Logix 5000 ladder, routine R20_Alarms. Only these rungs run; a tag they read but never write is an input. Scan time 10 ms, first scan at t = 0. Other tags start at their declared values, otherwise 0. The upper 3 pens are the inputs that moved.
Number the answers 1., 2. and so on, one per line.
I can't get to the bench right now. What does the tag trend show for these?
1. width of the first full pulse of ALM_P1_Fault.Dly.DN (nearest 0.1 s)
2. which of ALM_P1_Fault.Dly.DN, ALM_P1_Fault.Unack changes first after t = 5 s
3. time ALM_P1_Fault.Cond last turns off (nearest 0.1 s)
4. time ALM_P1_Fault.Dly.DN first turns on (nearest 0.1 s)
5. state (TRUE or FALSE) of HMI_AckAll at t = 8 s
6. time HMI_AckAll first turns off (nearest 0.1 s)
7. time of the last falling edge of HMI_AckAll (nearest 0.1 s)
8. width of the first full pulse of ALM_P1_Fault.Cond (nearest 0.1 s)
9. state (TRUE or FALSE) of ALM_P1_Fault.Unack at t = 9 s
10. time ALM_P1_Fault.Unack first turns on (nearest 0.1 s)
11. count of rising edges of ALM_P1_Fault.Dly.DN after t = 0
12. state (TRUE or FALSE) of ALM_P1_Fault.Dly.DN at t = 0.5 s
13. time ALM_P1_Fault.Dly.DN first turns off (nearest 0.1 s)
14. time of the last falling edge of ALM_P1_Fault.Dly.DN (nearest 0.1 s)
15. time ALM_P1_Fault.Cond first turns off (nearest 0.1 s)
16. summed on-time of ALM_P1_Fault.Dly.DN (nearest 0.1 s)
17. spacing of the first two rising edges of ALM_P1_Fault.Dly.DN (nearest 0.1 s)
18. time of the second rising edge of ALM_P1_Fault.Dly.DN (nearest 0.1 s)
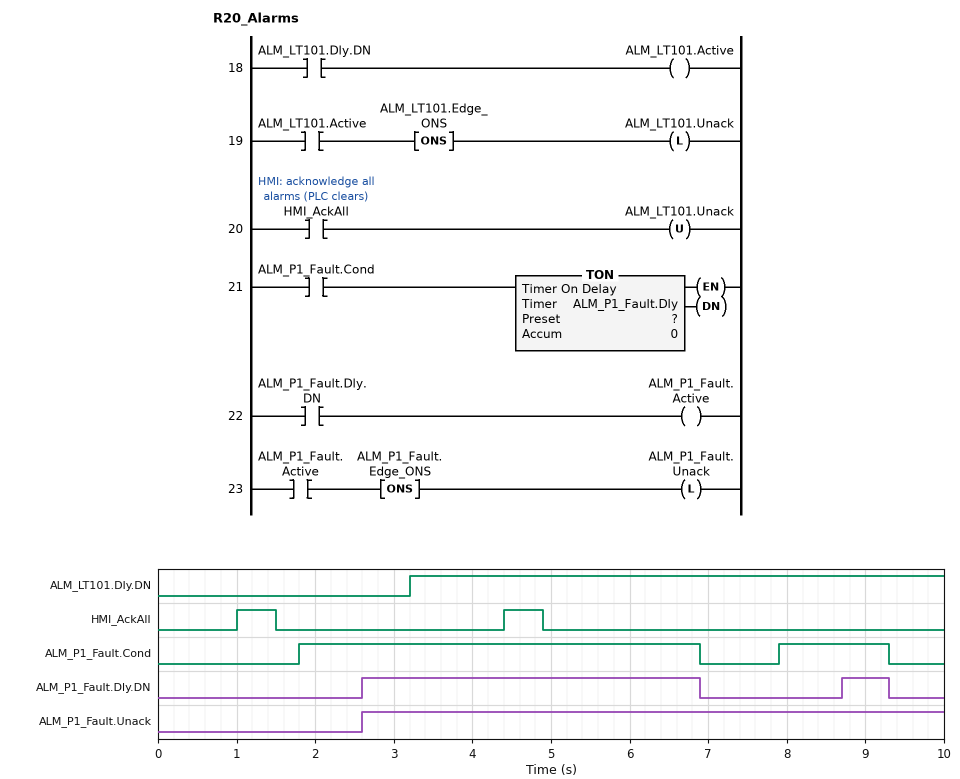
1. 4.3 s
2. ALM_P1_Fault.Dly.DN
3. 9.3 s
4. 2.6 s
5. FALSE
6. 1.5 s
7. 4.9 s
8. 5.1 s
9. TRUE
10. 2.6 s
11. 2
12. FALSE
13. 6.9 s
14. 9.3 s
15. 6.9 s
16. 4.9 s
17. 6.1 s
18. 8.7 s
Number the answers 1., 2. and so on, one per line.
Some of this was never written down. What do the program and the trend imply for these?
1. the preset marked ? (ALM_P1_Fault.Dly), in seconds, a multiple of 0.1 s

1. 0.8 s
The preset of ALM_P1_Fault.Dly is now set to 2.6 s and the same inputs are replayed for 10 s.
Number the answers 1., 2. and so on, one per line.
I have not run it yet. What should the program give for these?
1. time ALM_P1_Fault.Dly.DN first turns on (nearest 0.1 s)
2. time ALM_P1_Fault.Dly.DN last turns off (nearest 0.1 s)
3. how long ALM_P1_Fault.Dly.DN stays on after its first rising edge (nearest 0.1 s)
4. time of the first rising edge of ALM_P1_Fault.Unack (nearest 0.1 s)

1. 4.4 s
2. 6.9 s
3. 2.5 s
4. 4.4 s
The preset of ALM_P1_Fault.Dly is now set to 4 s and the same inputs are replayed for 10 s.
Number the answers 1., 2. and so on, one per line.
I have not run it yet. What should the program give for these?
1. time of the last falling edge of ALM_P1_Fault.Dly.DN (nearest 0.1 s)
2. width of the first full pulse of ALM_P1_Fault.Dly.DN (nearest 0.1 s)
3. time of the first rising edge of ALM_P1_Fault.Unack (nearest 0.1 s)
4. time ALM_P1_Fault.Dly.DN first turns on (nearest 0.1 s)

1. 6.9 s
2. 1.1 s
3. 5.8 s
4. 5.8 s
